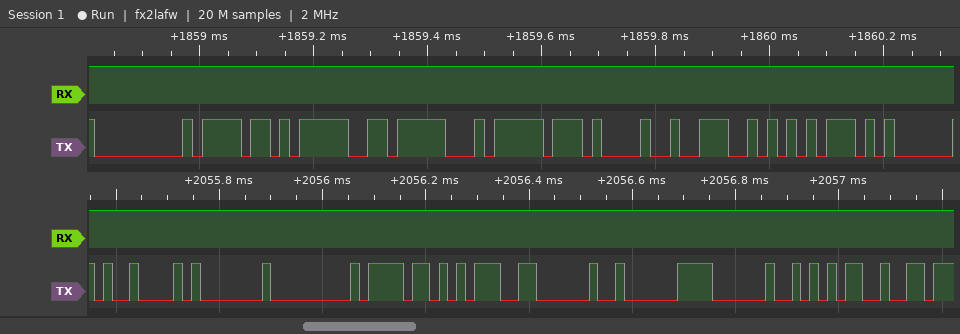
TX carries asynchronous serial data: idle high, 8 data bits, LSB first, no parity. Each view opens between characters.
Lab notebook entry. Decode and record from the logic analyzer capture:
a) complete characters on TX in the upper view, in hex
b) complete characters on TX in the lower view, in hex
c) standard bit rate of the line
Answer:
00, 6F, 9F, 1F, DF, 21, 4E, 75
09, 01, 00, 6F, 9D, 20, E0, 20, 35
57600 baud
